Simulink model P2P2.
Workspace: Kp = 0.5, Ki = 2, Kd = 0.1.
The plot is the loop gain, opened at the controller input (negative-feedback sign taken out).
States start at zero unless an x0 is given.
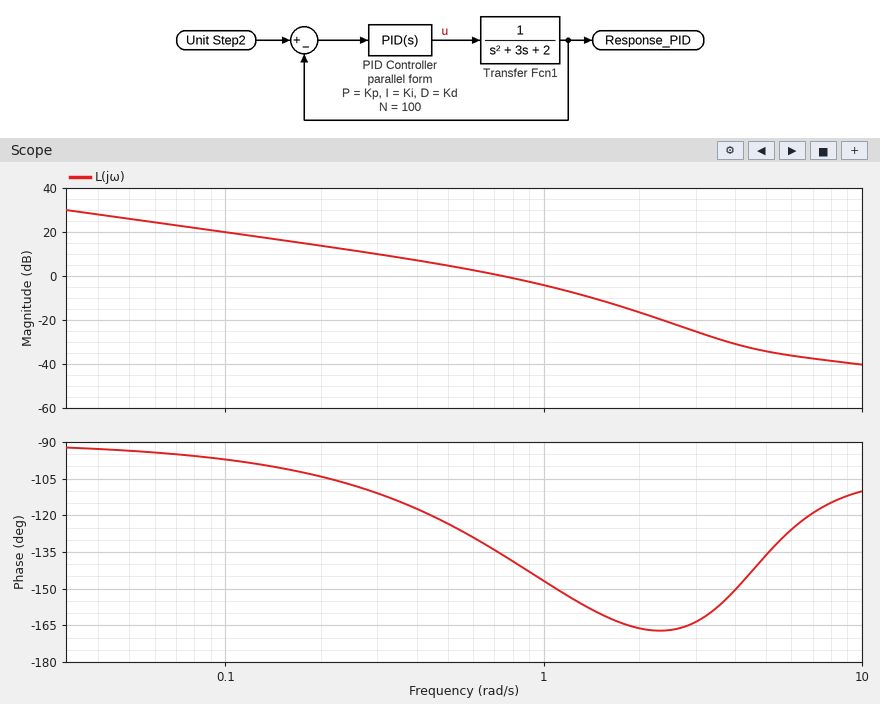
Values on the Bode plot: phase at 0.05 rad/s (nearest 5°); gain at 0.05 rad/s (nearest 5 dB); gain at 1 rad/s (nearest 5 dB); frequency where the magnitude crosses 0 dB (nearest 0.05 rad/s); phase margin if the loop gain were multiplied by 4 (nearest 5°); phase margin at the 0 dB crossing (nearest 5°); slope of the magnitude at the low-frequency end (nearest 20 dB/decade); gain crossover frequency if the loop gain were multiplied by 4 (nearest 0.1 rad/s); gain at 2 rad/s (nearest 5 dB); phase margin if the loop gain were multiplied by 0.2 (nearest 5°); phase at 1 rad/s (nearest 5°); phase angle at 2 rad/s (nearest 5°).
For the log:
-95°
25 dB
-5 dB
0.75 rad/s
20°
45°
-20 dB/decade
1.6 rad/s
-15 dB
75°
-145°
-165°
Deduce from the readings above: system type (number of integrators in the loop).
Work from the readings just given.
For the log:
1
